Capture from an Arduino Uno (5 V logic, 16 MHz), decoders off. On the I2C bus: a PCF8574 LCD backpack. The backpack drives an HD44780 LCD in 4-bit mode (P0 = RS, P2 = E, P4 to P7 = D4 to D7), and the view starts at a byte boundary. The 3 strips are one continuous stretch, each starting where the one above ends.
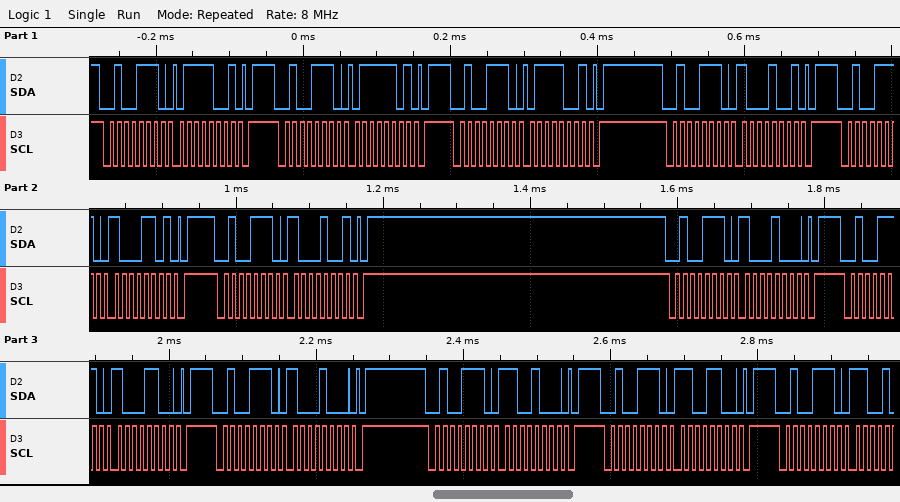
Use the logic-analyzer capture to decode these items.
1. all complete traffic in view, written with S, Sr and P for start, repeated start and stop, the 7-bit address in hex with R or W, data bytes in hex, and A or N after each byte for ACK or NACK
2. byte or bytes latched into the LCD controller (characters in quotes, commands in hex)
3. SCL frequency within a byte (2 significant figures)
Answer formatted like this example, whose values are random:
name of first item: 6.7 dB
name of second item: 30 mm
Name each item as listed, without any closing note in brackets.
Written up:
all complete traffic in view, written with S, Sr and P for start, repeated start and stop, the 7-bit address in hex with R or W, data bytes in hex, and A or N after each byte for ACK or NACK: S 27W A 79 A P S 27W A 7D A P S 27W A 79 A P S 27W A 89 A P S 27W A 8D A P S 27W A 89 A P S 27W A 88 A P S 27W A 8C A P S 27W A 88 A P S 27W A C8 A P S 27W A CC A P S 27W A
byte or bytes latched into the LCD controller: 'x'
SCL frequency within a byte: 100 kHz
